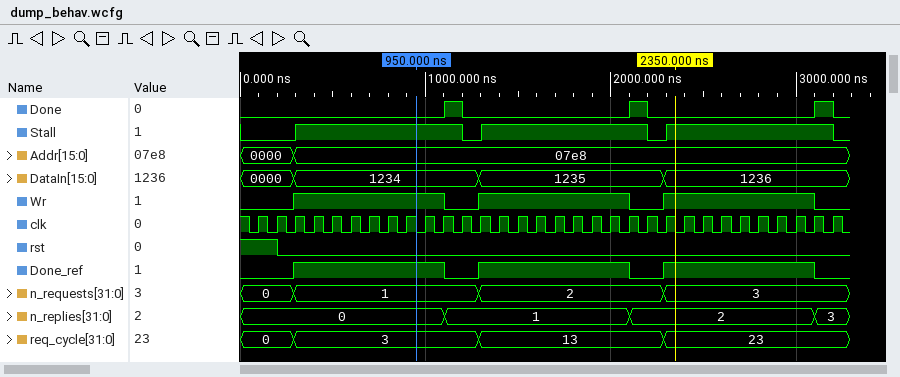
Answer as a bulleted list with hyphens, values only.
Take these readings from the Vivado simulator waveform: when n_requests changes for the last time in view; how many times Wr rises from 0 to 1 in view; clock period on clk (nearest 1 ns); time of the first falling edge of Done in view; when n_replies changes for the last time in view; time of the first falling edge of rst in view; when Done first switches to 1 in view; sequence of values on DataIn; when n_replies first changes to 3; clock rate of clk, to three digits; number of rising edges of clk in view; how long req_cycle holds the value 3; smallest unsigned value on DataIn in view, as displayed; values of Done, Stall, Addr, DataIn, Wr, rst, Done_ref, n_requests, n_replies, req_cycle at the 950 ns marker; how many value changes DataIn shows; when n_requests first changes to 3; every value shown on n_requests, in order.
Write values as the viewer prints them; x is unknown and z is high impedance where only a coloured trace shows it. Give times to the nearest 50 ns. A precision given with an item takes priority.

- 2300 ns
- 3
- 100 ns
- 1200 ns
- 3100 ns
- 200 ns
- 1100 ns
- 0000, 1234, 1235, 1236
- 3100 ns
- 10.0 MHz
- 32
- 1000 ns
- 0000
- Done=0, Stall=1, Addr=07e8, DataIn=1234, Wr=1, rst=0, Done_ref=1, n_requests=1, n_replies=0, req_cycle=3
- 3
- 2300 ns
- 0, 1, 2, 3
